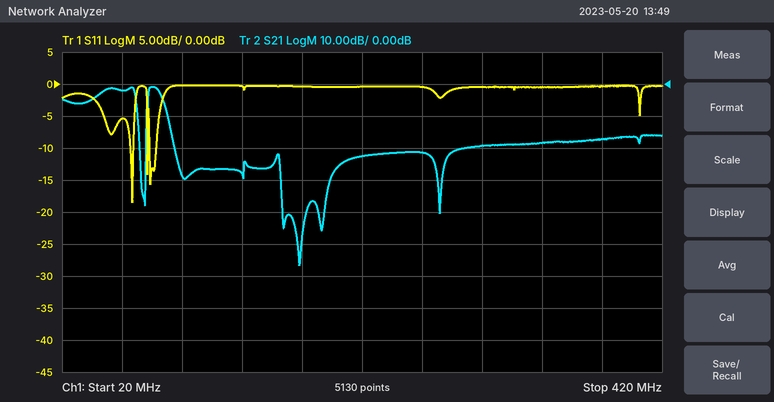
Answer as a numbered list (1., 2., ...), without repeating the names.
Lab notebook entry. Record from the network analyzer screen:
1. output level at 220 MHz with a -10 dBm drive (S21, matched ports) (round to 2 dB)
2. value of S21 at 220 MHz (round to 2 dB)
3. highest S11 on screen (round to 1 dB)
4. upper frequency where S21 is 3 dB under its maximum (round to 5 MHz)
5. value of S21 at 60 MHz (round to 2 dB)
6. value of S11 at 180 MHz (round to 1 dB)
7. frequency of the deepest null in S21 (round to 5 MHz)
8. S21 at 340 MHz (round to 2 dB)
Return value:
1. -32 dBm
2. -22 dB
3. 0 dB
4. 85 MHz
5. -2 dB
6. 0 dB
7. 180 MHz
8. -18 dB
